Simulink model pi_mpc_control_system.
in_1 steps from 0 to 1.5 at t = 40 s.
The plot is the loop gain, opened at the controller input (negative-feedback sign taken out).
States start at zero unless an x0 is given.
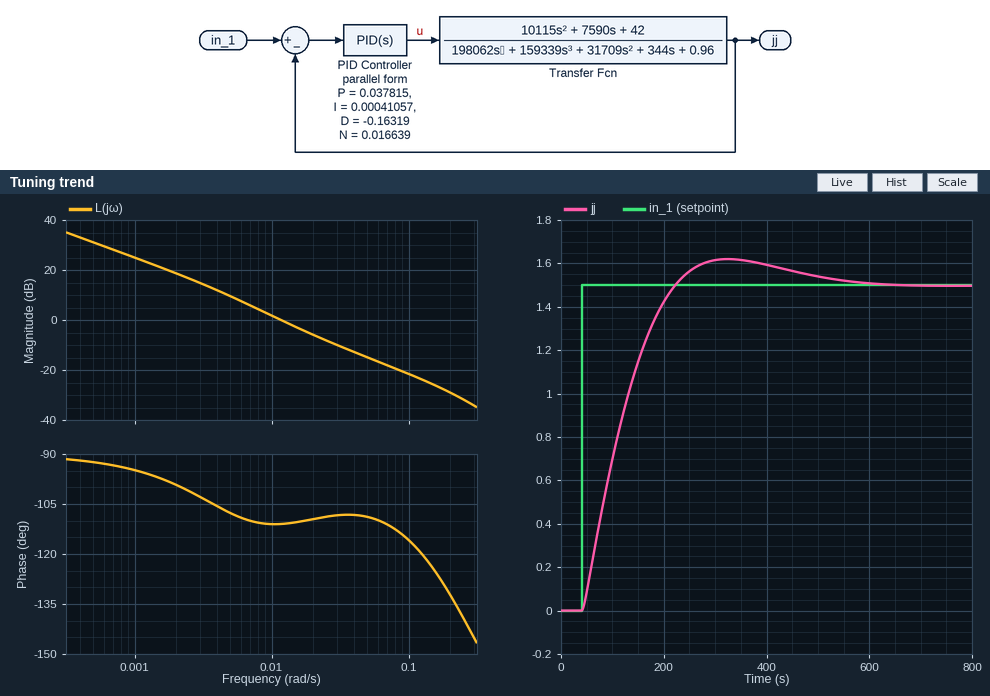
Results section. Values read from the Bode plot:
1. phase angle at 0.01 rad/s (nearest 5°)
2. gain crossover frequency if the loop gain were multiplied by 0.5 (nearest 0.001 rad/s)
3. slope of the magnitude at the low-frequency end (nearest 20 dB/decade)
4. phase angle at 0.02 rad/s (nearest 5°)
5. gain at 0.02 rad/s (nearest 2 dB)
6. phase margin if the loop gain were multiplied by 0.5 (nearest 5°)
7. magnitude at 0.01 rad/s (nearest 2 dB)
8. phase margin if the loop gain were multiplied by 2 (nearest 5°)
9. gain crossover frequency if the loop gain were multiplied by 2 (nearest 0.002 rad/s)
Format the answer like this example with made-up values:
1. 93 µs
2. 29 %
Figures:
1. -110°
2. 0.007 rad/s
3. -20 dB/decade
4. -110°
5. -6 dB
6. 70°
7. 2 dB
8. 70°
9. 0.020 rad/s
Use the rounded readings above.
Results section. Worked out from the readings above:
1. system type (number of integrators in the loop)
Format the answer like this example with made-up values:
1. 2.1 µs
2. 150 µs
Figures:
1. 1
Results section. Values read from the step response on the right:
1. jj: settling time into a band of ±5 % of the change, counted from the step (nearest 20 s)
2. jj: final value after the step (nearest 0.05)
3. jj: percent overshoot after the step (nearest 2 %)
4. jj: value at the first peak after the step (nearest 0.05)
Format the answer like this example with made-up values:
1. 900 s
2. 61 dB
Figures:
1. 400 s
2. 1.50
3. 8 %
4. 1.60
